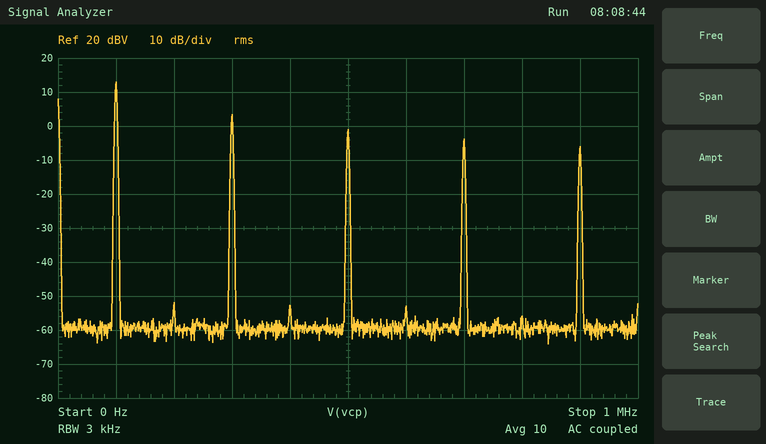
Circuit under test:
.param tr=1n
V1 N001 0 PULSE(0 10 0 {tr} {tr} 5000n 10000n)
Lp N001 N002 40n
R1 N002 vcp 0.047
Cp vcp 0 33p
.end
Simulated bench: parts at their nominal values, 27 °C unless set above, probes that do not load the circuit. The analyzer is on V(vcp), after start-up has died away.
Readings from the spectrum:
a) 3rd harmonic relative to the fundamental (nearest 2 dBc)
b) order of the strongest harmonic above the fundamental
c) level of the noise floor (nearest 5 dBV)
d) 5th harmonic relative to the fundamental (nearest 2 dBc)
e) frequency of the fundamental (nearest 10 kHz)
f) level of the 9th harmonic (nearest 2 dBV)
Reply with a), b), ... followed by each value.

a) -10 dBc
b) 3
c) -60 dBV
d) -14 dBc
e) 100 kHz
f) -6 dBV
